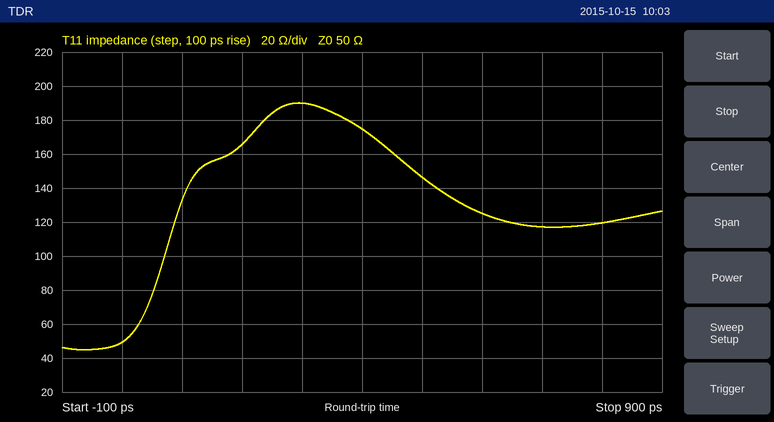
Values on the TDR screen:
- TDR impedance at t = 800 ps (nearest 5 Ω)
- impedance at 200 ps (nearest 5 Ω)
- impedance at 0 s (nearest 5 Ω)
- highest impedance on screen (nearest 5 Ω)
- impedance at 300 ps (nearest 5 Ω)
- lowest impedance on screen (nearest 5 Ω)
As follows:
120 Ω
165 Ω
50 Ω
190 Ω
190 Ω
45 Ω
